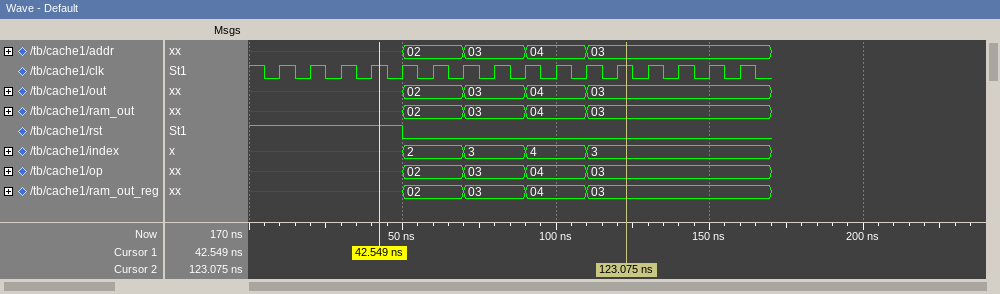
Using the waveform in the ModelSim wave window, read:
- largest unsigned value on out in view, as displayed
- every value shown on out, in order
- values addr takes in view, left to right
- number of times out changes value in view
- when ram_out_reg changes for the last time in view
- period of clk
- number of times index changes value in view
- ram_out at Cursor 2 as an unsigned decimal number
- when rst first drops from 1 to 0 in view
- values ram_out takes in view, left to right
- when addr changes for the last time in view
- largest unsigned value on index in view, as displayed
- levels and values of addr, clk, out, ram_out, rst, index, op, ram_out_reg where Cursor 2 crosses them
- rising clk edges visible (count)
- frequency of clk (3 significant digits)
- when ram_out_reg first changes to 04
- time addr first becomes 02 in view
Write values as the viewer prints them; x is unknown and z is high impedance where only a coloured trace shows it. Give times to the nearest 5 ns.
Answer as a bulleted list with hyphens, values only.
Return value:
- 04
- x, 02, 03, 04, 03
- x, 02, 03, 04, 03
- 4
- 110 ns
- 10 ns
- 4
- 3
- 50 ns
- x, 02, 03, 04, 03
- 110 ns
- 4
- addr=03, clk=1, out=03, ram_out=03, rst=0, index=3, op=03, ram_out_reg=03
- 16
- 100 MHz
- 90 ns
- 50 ns
